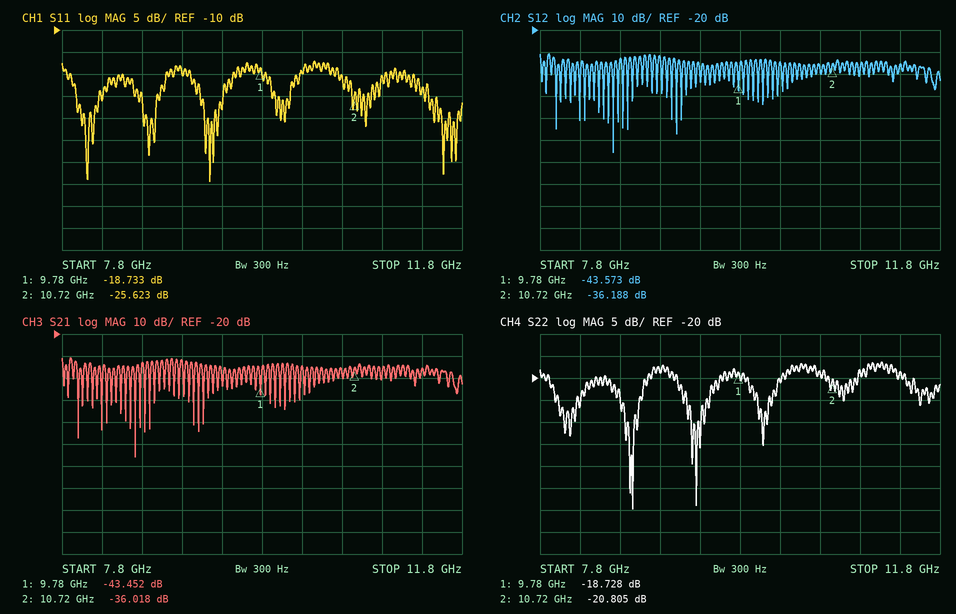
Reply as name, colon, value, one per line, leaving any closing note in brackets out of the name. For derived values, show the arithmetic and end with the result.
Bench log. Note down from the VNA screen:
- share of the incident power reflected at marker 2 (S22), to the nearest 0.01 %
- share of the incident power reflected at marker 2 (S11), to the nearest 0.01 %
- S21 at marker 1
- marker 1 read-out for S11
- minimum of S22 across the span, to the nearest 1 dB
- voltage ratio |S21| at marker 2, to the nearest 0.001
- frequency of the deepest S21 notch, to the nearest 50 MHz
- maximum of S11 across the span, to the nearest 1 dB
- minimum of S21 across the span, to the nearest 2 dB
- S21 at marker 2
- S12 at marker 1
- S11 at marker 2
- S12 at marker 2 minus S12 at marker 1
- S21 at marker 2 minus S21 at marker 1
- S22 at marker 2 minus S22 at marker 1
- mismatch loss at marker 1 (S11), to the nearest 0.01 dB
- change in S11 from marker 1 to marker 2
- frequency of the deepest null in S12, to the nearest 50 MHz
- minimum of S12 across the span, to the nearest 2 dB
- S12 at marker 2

share of the incident power reflected at marker 2 (S22), to the nearest 0.01 %: 10^(-20.805/10) ≈ 0.83 %
share of the incident power reflected at marker 2 (S11), to the nearest 0.01 %: 10^(-25.623/10) ≈ 0.27 %
S21 at marker 1: -43.452 dB
marker 1 read-out for S11: -18.733 dB
minimum of S22 across the span, to the nearest 1 dB: -50 dB
voltage ratio |S21| at marker 2, to the nearest 0.001: 10^(-36.018/20) ≈ 0.016
frequency of the deepest S21 notch, to the nearest 50 MHz: 8.55 GHz
maximum of S11 across the span, to the nearest 1 dB: -17 dB
minimum of S21 across the span, to the nearest 2 dB: -76 dB
S21 at marker 2: -36.018 dB
S12 at marker 1: -43.573 dB
S11 at marker 2: -25.623 dB
S12 at marker 2 minus S12 at marker 1: -36.188 − (-43.573) = 7.385 dB
S21 at marker 2 minus S21 at marker 1: -36.018 − (-43.452) = 7.434 dB
S22 at marker 2 minus S22 at marker 1: -20.805 − (-18.728) = -2.077 dB
mismatch loss at marker 1 (S11), to the nearest 0.01 dB: −10 log10(1 − 10^(-18.733/10)) ≈ 0.06 dB
change in S11 from marker 1 to marker 2: -25.623 − (-18.733) = -6.890 dB
frequency of the deepest null in S12, to the nearest 50 MHz: 8.55 GHz
minimum of S12 across the span, to the nearest 2 dB: -76 dB
S12 at marker 2: -36.188 dB
